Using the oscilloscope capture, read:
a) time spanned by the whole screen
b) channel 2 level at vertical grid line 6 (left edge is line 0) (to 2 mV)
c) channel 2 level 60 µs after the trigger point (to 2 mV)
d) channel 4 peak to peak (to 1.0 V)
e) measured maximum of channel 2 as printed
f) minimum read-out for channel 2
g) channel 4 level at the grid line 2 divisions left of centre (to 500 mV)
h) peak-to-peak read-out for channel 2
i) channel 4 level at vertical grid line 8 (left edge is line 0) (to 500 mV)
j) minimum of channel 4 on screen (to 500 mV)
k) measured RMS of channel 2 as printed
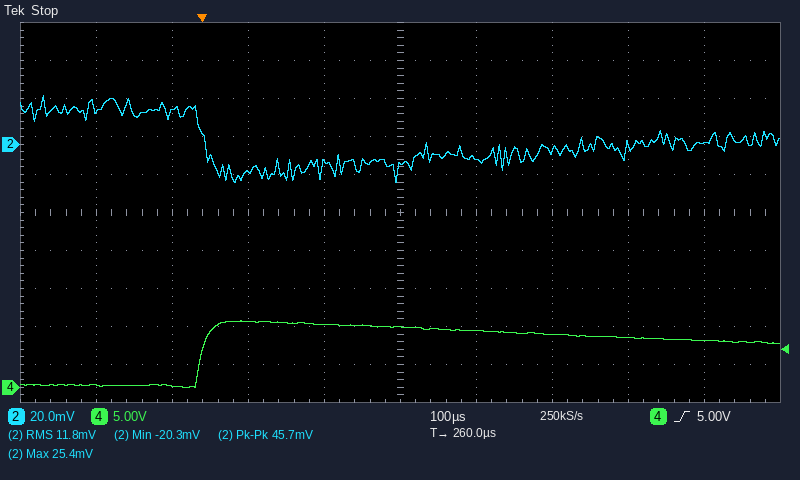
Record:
1 ms
-8 mV
-14 mV
9.0 V
25.4 mV
-20.3 mV
8.5 V
45.7 mV
6.5 V
0.0 V
11.8 mV
